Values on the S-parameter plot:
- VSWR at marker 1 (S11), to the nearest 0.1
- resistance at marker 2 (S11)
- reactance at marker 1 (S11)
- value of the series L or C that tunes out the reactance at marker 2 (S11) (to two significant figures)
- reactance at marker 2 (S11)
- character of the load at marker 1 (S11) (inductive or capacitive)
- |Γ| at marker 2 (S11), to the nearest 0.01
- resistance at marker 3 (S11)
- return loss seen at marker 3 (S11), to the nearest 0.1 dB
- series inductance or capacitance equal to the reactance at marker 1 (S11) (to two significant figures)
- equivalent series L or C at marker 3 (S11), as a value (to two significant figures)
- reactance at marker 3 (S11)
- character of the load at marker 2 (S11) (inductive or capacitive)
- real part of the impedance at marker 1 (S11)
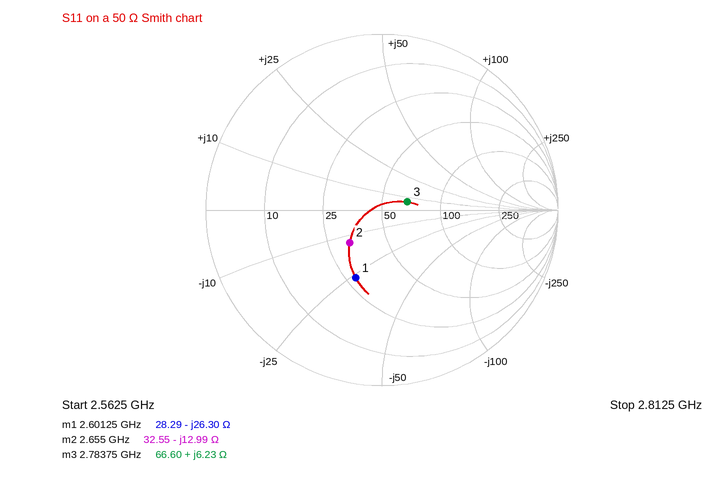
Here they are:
2.4
32.55 Ω
-26.30 Ω
780 pH
-12.99 Ω
capacitive
0.26
66.60 Ω
16.4 dB
2.3 pF
360 pH
+6.23 Ω
capacitive
28.29 Ω
